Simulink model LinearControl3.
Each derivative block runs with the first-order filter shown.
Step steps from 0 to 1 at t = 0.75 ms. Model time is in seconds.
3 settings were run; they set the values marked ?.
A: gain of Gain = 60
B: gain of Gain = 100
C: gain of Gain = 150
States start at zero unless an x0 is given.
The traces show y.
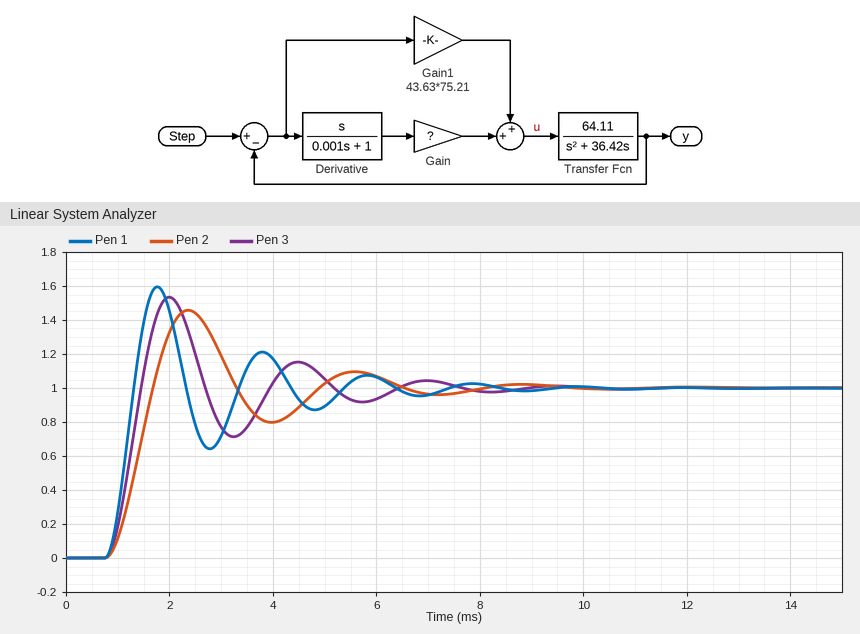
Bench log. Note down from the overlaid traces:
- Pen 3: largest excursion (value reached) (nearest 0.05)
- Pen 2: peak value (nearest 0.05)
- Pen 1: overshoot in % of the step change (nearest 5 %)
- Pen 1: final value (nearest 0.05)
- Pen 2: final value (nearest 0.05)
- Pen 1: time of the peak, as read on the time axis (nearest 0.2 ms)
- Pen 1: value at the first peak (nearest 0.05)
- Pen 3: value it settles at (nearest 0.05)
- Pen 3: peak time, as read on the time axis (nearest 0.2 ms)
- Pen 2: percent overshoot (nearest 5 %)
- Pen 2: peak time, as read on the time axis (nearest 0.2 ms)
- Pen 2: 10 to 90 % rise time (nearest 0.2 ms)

1.55
1.45
60 %
1.00
1.00
1.8 ms
1.60
1.00
2.0 ms
45 %
2.4 ms
0.6 ms
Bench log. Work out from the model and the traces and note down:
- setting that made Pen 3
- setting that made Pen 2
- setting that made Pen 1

B
A
C
